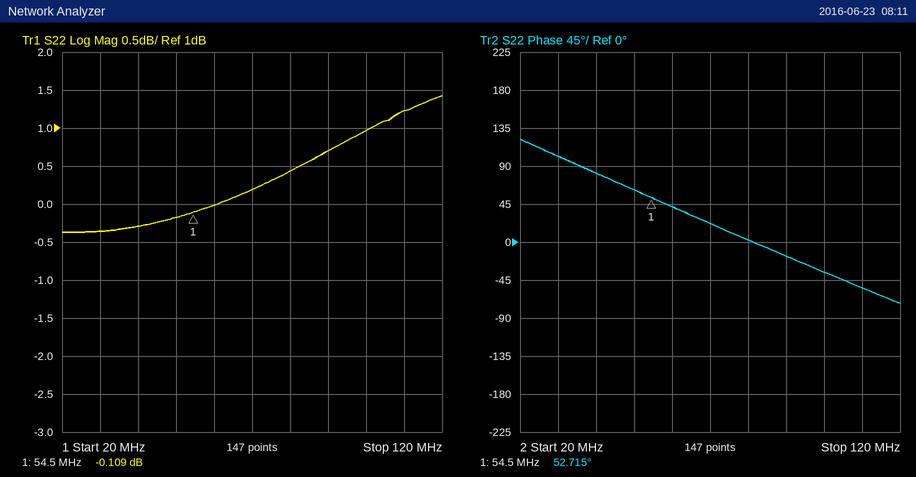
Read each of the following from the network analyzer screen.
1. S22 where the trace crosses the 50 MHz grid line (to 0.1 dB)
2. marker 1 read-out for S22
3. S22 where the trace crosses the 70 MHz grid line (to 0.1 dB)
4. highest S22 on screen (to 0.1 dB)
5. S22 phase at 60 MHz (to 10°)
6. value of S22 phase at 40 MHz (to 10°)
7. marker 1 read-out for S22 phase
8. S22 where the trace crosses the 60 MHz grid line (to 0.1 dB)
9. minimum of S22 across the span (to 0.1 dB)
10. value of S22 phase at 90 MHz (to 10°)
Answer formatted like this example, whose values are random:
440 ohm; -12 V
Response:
-0.2 dB; -0.109 dB; 0.2 dB; 1.4 dB; 40°; 80°; 52.715°; 0.0 dB; -0.4 dB; -20°
